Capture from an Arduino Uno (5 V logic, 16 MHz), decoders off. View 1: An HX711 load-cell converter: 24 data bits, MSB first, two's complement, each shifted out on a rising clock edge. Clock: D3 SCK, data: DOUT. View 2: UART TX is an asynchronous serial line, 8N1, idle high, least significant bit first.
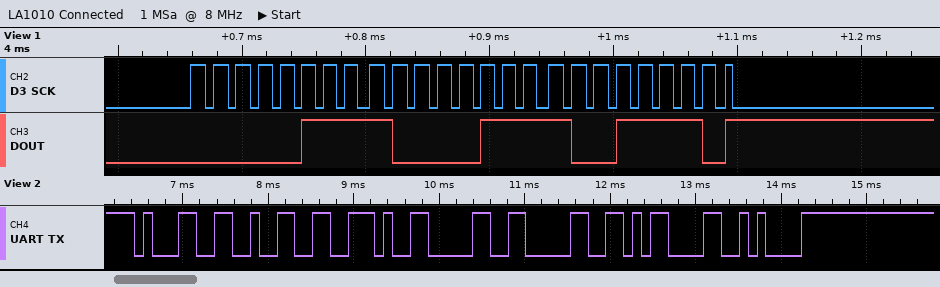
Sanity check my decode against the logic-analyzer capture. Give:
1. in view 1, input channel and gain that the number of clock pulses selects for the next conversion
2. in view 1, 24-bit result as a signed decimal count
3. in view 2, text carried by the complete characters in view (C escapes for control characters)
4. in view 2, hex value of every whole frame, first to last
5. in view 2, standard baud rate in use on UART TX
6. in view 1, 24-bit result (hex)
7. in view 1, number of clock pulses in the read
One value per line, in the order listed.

channel A, gain 128
493470
"12.00\r\n"
31 32 2E 30 30 0D 0A
9600 baud
0x07879E
25
